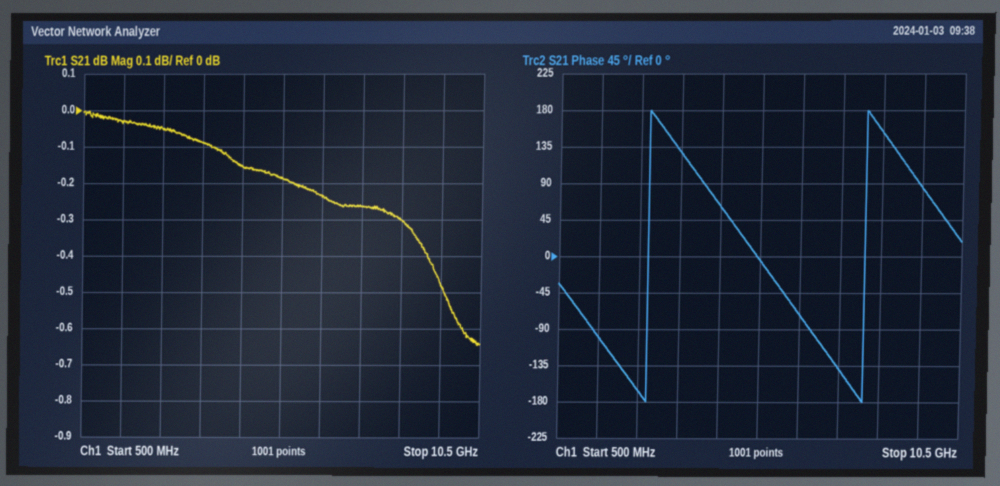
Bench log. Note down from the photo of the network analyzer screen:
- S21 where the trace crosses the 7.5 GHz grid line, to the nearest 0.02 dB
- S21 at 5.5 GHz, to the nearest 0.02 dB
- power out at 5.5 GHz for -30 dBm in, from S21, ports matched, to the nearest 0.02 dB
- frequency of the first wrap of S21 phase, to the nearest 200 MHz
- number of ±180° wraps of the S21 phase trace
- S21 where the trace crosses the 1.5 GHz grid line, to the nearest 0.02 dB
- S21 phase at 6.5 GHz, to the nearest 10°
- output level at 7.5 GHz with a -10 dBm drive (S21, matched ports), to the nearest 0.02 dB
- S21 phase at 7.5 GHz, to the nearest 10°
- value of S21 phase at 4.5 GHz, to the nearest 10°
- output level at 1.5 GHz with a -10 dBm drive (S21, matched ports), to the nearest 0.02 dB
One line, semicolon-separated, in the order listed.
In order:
-0.26 dB; -0.18 dB; -30.18 dBm; 2.8 GHz; 2; -0.02 dB; -70°; -10.26 dBm; -140°; 60°; -10.02 dBm
